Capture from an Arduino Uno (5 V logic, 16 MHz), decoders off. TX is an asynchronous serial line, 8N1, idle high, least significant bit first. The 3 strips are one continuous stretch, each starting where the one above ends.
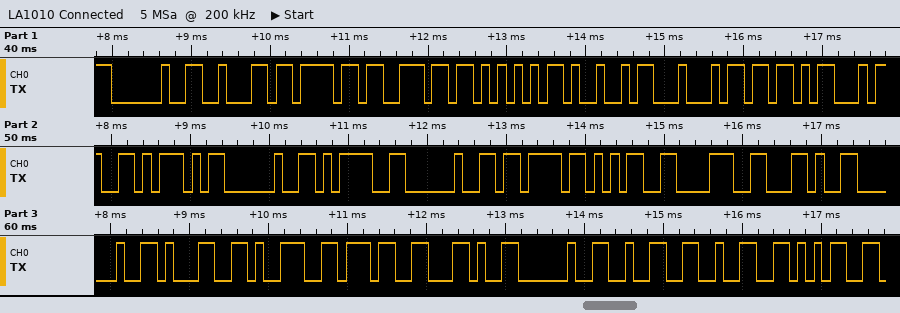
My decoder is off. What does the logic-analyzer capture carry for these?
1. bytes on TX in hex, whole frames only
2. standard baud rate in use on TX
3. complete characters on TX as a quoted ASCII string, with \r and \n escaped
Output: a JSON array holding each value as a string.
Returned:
["20 62 6F 6E 55 49 44 5B 34 5D 20 3D 20 7B 35 38 2C 20 31 39 37 2C 20 32 32 35", "9600 baud", "\" bonUID[4] = {58, 197, 225\""]
